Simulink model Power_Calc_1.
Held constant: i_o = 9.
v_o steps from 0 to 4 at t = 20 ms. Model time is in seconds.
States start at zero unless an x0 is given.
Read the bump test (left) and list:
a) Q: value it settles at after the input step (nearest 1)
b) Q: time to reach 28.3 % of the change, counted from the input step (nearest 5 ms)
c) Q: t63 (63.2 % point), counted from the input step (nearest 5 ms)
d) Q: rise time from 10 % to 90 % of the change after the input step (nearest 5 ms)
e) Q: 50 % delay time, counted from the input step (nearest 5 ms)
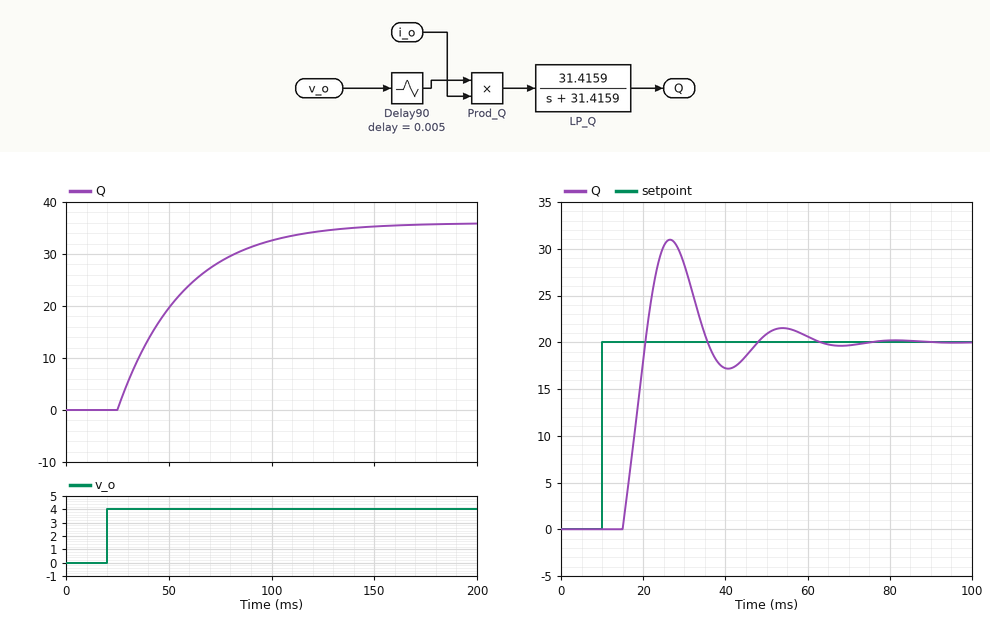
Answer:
36
15 ms
35 ms
70 ms
25 ms
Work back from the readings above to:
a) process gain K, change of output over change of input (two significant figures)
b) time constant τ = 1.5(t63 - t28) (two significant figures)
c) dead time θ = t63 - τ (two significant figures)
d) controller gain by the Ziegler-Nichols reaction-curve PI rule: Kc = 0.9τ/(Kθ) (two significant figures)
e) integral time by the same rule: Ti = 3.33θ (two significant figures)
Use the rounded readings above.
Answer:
9.0
30 ms
5.0 ms
0.60
17 ms
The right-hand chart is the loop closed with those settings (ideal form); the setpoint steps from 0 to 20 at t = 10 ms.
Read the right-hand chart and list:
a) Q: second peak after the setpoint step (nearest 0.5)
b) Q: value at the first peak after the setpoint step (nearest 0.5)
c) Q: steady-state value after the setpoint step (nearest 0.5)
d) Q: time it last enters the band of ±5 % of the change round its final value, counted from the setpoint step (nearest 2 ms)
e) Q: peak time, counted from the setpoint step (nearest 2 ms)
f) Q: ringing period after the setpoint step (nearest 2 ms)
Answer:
21.5
31.0
20.0
48 ms
16 ms
28 ms
